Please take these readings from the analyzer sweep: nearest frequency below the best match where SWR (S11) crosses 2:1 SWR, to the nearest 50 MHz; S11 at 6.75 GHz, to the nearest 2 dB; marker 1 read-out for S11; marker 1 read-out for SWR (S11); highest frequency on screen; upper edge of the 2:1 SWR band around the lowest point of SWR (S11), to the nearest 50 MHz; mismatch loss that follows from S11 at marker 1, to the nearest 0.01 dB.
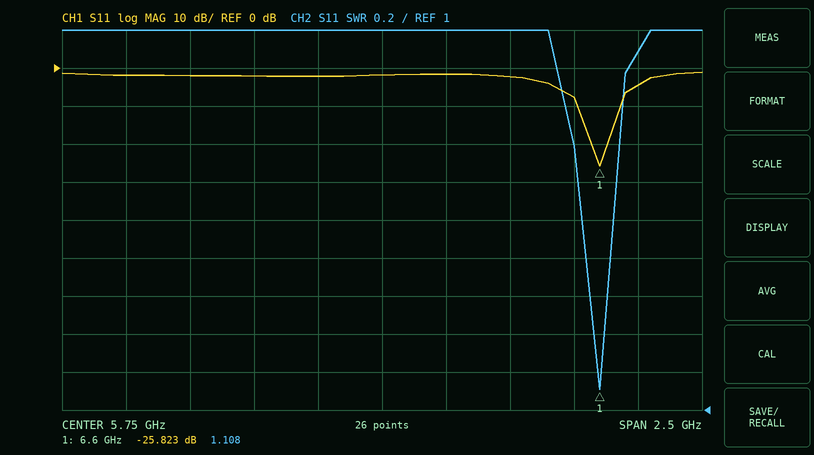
6.55 GHz
-4 dB
-25.823 dB
1.108
7 GHz
6.65 GHz
0.01 dB
